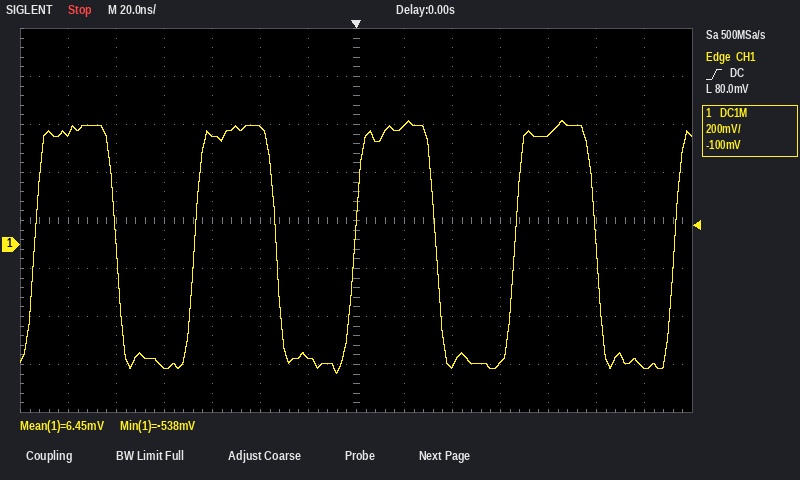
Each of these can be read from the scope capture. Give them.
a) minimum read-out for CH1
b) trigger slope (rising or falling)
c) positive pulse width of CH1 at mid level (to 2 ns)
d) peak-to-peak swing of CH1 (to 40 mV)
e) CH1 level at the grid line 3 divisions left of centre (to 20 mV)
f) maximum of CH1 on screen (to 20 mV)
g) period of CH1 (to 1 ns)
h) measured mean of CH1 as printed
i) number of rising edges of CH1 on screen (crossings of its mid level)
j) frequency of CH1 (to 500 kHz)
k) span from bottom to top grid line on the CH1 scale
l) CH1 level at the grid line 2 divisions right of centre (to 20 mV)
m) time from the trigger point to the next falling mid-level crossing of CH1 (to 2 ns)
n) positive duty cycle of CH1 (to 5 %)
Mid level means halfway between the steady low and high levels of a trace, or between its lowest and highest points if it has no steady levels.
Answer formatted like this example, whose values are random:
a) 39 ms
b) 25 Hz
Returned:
a) -538 mV
b) rising
c) 34 ns
d) 1.04 V
e) 460 mV
f) 520 mV
g) 67 ns
h) 6.45 mV
i) 5
j) 15.0 MHz
k) 1.6 V
l) -500 mV
m) 34 ns
n) 50 %
